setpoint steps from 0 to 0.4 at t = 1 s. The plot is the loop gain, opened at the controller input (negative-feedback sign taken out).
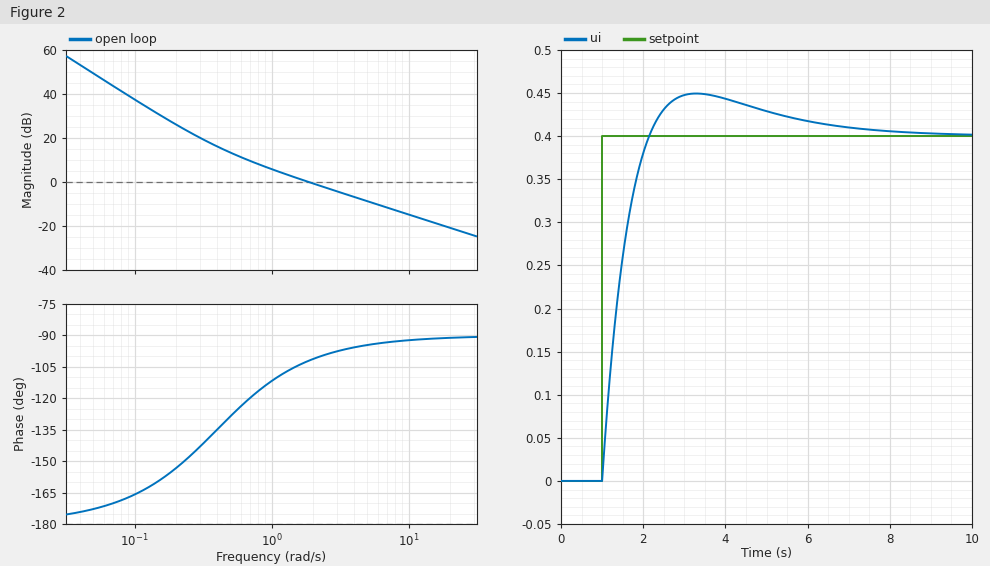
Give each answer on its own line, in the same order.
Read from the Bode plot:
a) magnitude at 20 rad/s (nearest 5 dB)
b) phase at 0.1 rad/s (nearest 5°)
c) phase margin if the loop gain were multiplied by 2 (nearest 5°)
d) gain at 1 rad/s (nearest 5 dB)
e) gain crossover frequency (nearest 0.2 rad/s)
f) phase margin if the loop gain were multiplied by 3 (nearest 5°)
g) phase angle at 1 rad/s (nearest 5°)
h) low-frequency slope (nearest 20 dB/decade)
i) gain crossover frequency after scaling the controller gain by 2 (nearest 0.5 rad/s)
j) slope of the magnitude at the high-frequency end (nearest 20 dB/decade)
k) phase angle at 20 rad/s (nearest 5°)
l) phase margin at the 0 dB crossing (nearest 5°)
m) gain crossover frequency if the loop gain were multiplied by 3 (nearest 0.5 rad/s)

-20 dB
-165°
85°
5 dB
1.8 rad/s
85°
-110°
-40 dB/decade
3.5 rad/s
-20 dB/decade
-90°
80°
5.5 rad/s
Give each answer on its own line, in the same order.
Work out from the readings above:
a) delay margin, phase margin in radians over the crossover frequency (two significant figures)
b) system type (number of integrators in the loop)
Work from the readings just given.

0.78 s
2
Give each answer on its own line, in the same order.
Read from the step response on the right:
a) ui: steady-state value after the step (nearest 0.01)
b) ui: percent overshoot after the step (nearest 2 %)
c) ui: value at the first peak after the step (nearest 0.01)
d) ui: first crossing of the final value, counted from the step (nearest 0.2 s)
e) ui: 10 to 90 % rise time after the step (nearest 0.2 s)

0.40
12 %
0.45
1.2 s
0.8 s
